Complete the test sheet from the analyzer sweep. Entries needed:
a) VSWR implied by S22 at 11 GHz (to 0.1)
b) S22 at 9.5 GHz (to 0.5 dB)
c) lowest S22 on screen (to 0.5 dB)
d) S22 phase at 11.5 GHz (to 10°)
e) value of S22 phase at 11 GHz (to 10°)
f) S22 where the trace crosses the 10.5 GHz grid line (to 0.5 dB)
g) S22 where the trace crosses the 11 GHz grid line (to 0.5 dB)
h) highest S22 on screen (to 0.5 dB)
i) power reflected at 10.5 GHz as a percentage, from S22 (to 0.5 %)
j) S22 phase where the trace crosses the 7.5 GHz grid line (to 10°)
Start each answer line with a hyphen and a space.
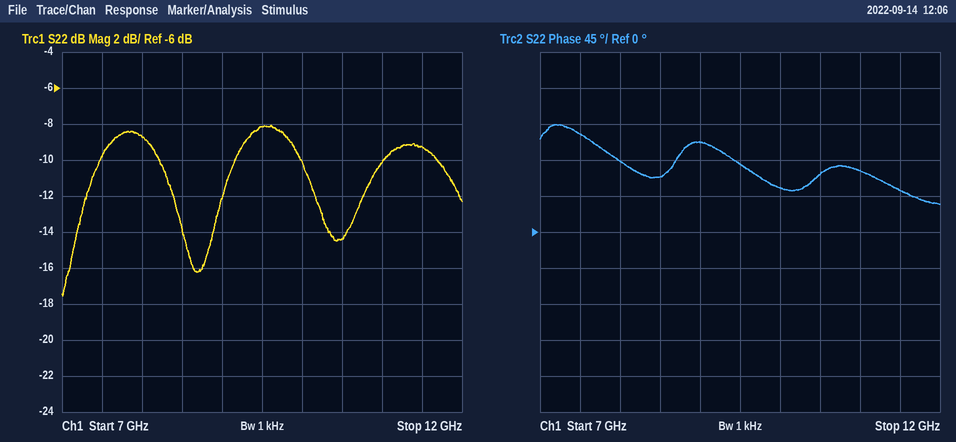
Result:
- 1.9
- -8.0 dB
- -17.5 dB
- 50°
- 80°
- -14.5 dB
- -10.0 dB
- -8.0 dB
- 3.5 %
- 120°
